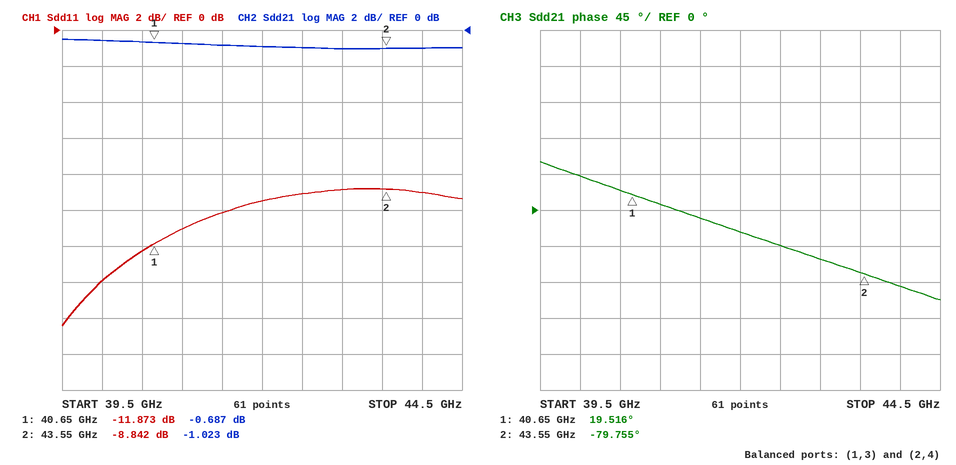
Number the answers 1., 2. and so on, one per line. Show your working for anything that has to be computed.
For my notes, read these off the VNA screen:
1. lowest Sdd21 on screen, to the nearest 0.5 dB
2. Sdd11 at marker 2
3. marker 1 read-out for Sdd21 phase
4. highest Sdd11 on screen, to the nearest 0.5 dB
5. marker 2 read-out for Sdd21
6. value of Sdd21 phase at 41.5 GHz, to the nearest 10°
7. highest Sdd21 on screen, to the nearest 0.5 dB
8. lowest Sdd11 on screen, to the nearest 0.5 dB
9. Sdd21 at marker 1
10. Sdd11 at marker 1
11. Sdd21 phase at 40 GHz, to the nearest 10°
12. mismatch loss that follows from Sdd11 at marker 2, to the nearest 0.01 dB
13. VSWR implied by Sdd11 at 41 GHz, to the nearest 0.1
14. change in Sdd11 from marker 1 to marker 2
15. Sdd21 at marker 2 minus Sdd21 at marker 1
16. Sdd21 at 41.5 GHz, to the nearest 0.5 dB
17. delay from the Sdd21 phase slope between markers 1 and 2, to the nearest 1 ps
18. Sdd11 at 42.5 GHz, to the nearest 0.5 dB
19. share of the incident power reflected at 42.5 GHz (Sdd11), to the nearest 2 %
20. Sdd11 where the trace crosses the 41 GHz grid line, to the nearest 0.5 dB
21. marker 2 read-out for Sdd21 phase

1. -1.0 dB
2. -8.842 dB
3. 19.516°
4. -9.0 dB
5. -1.023 dB
6. -10°
7. -0.5 dB
8. -16.5 dB
9. -0.687 dB
10. -11.873 dB
11. 40°
12. −10 log10(1 − 10^(-8.842/10)) ≈ 0.61 dB
13. |Γ| = 10^(-11/20) = 0.2818; VSWR = (1 + 0.2818)/(1 − 0.2818) ≈ 1.8
14. -8.842 − (-11.873) = 3.031 dB
15. -1.023 − (-0.687) = -0.336 dB
16. -1.0 dB
17. −(-79.755° − (19.516°))/(360° × 2.9 GHz) ≈ 95 ps
18. -9.0 dB
19. 10^(-9/10) ≈ 12.6 %, so 12 % to the nearest 2 %
20. -11.0 dB
21. -79.755°
